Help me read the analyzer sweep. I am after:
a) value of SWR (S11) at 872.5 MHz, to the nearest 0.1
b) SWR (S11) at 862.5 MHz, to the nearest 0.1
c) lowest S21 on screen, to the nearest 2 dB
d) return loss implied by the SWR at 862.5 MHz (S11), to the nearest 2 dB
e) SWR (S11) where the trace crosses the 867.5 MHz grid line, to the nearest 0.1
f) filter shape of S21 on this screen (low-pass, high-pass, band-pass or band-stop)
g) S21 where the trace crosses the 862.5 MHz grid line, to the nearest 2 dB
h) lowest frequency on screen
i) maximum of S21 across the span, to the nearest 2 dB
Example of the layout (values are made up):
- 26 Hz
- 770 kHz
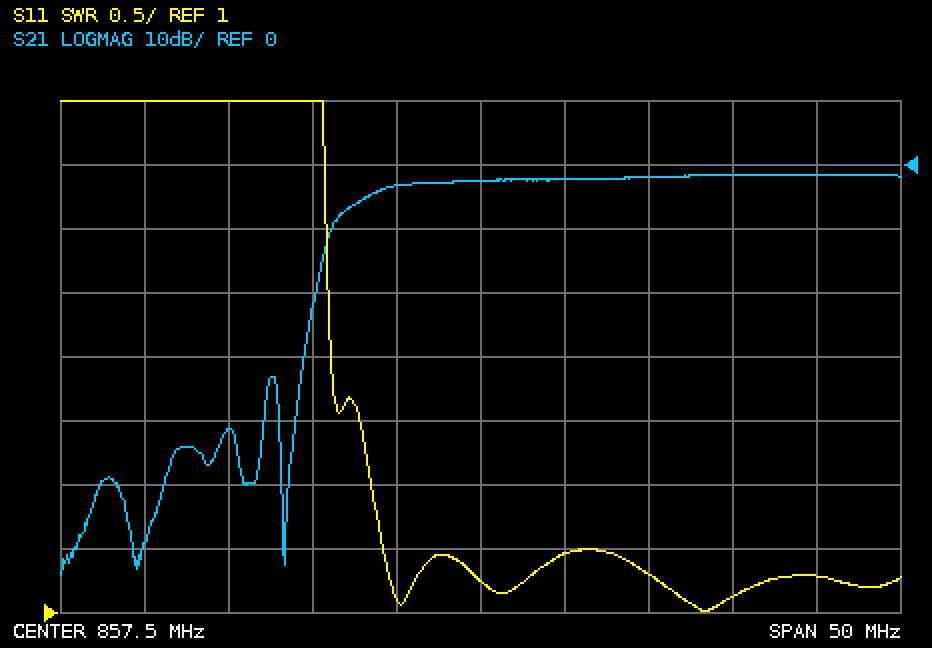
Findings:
- 1.1
- 1.5
- -64 dB
- 14 dB
- 1.3
- high-pass
- -2 dB
- 832.5 MHz
- -2 dB
